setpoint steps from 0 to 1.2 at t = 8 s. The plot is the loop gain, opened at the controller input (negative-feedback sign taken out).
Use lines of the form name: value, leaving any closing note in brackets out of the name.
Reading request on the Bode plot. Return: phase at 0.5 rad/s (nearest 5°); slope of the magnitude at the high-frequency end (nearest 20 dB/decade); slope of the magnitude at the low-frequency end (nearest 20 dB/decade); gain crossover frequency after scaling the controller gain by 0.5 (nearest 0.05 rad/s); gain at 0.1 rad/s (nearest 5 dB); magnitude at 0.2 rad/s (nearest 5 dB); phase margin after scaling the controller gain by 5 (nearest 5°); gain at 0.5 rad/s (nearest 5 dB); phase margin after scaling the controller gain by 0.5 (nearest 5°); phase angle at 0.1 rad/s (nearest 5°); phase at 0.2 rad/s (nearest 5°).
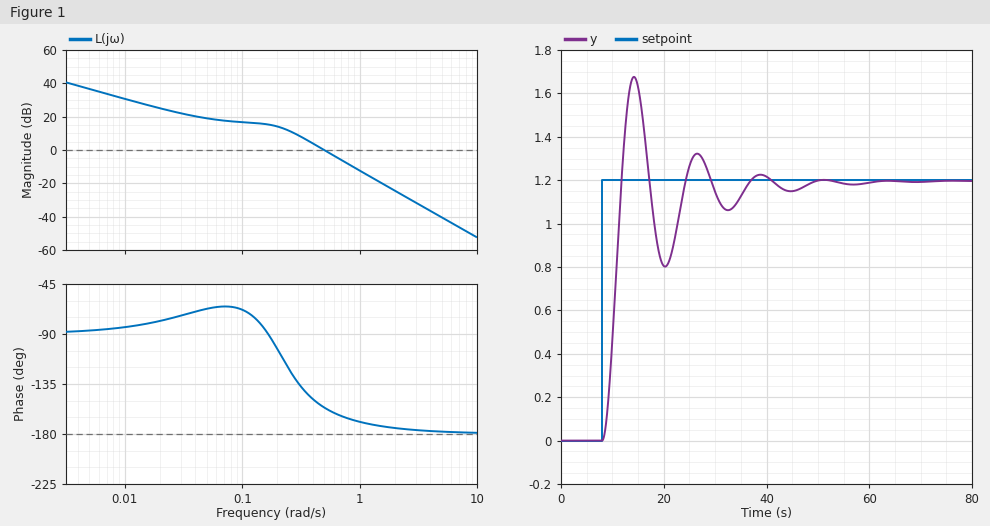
phase at 0.5 rad/s: -155°
slope of the magnitude at the high-frequency end: -40 dB/decade
slope of the magnitude at the low-frequency end: -20 dB/decade
gain crossover frequency after scaling the controller gain by 0.5: 0.35 rad/s
gain at 0.1 rad/s: 15 dB
magnitude at 0.2 rad/s: 15 dB
phase margin after scaling the controller gain by 5: 10°
gain at 0.5 rad/s: 0 dB
phase margin after scaling the controller gain by 0.5: 35°
phase angle at 0.1 rad/s: -70°
phase at 0.2 rad/s: -105°
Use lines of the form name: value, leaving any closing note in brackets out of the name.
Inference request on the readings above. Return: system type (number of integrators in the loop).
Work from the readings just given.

system type: 1
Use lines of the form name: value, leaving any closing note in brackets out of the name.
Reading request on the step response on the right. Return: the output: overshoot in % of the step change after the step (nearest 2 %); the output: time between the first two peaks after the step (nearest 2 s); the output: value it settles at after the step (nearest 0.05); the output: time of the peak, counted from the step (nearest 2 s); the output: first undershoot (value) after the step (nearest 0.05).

the output: overshoot in % of the step change after the step: 40 %
the output: time between the first two peaks after the step: 12 s
the output: value it settles at after the step: 1.20
the output: time of the peak, counted from the step: 6 s
the output: first undershoot (value) after the step: 0.80
